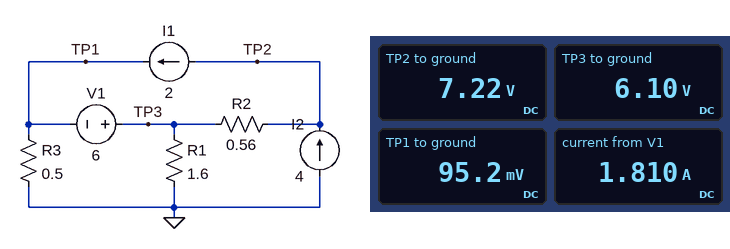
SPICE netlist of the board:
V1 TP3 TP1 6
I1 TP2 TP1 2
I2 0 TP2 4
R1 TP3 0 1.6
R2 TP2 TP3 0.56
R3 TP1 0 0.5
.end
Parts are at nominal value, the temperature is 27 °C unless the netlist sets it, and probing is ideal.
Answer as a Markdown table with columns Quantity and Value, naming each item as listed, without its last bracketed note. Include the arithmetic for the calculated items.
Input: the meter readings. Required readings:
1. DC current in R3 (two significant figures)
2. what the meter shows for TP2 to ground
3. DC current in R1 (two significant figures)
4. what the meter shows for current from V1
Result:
| Quantity | Value |
|---|---|
| DC current in R3 | (95.2 mV) / 500 mΩ = 190 mA |
| what the meter shows for TP2 to ground | 7.22 V |
| DC current in R1 | (6.1 V) / 1.6 Ω = 3.8 A |
| what the meter shows for current from V1 | 1.810 A |
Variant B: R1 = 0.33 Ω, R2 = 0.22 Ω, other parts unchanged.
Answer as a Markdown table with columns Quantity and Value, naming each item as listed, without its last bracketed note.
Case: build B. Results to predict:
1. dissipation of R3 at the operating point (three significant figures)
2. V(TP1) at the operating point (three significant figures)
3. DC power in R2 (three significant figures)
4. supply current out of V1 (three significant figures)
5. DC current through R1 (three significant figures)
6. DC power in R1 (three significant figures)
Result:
| Quantity | Value |
|---|---|
| dissipation of R3 at the operating point | 15.9 W |
| V(TP1) at the operating point | -2.82 V |
| DC power in R2 | 880 mW |
| supply current out of V1 | 7.64 A |
| DC current through R1 | 9.64 A |
| DC power in R1 | 30.7 W |
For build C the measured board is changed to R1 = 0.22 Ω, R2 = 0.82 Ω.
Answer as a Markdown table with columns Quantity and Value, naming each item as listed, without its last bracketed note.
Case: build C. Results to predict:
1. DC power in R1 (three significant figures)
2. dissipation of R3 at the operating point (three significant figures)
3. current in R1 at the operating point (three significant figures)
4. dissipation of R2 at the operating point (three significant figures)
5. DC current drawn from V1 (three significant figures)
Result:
| Quantity | Value |
|---|---|
| DC power in R1 | 27.2 W |
| dissipation of R3 at the operating point | 25.3 W |
| current in R1 at the operating point | 11.1 A |
| dissipation of R2 at the operating point | 3.28 W |
| DC current drawn from V1 | 9.11 A |
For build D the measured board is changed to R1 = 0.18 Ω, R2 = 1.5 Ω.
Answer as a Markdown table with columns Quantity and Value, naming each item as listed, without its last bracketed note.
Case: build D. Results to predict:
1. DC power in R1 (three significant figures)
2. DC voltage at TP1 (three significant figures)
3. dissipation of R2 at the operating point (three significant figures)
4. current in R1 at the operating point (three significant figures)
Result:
| Quantity | Value |
|---|---|
| DC power in R1 | 24.9 W |
| DC voltage at TP1 | -3.88 V |
| dissipation of R2 at the operating point | 6.00 W |
| current in R1 at the operating point | 11.8 A |
